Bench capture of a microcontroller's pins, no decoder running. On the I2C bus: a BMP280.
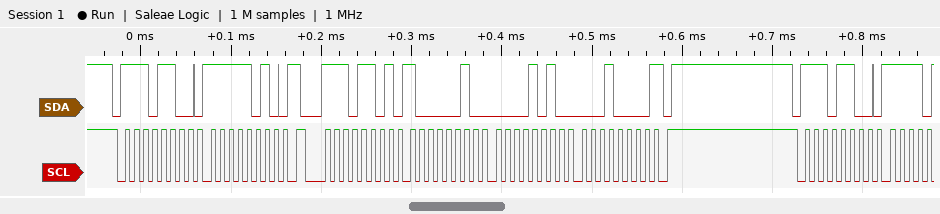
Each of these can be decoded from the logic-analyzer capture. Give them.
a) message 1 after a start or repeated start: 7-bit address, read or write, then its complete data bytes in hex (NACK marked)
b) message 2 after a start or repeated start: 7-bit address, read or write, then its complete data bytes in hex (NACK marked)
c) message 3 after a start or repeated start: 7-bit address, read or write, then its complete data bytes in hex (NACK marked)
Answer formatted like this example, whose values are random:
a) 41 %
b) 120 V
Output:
a) 0x76 write: FA
b) 0x76 read: 82 0A 10 NACK
c) 0x76 write
